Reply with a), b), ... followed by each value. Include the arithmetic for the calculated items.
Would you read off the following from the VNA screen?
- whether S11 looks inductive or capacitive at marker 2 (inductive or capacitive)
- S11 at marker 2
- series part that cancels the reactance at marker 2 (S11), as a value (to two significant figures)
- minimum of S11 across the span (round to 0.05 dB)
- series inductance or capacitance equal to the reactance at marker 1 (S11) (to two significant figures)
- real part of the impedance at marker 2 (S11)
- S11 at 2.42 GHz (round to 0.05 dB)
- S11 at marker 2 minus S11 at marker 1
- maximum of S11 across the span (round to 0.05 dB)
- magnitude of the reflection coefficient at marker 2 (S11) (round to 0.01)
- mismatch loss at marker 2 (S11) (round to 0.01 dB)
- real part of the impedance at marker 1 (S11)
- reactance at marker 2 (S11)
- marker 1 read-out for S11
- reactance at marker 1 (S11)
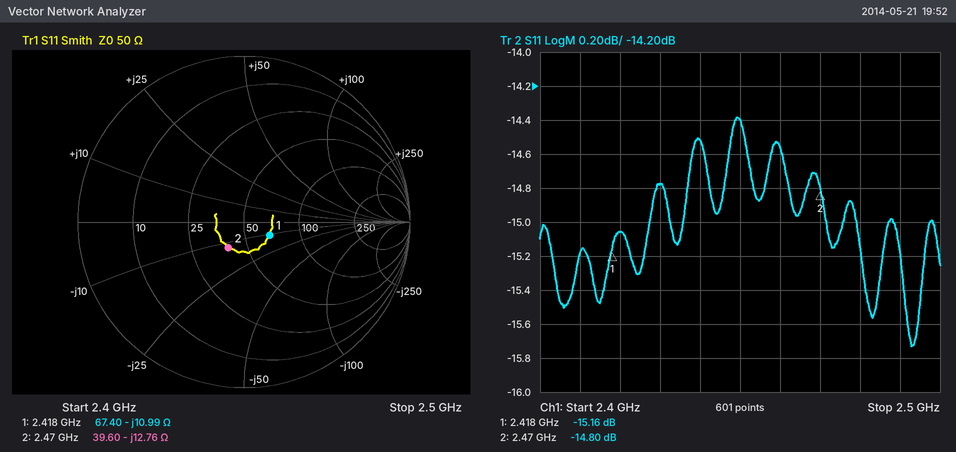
a) capacitive
b) -14.80 dB
c) L = 12.76 Ω/(2π × 2.47 GHz) ≈ 822 pH, so 820 pH to two significant figures
d) -15.75 dB
e) C = 1/(2π × 2.418 GHz × 10.99 Ω) ≈ 6.0 pF
f) 39.60 Ω
g) -15.05 dB
h) -14.8 − (-15.16) = 0.36 dB
i) -14.40 dB
j) 0.18
k) −10 log10(1 − 10^(-14.8/10)) ≈ 0.15 dB
l) 67.40 Ω
m) -12.76 Ω
n) -15.16 dB
o) -10.99 Ω
